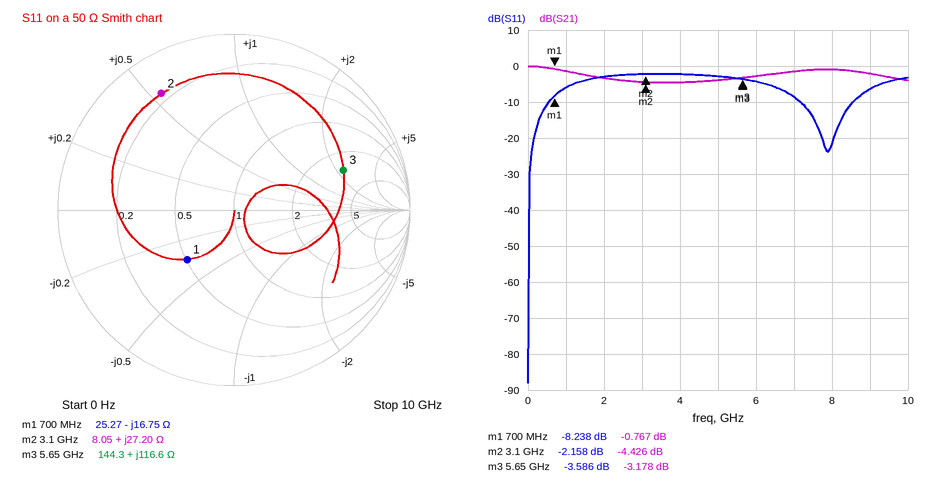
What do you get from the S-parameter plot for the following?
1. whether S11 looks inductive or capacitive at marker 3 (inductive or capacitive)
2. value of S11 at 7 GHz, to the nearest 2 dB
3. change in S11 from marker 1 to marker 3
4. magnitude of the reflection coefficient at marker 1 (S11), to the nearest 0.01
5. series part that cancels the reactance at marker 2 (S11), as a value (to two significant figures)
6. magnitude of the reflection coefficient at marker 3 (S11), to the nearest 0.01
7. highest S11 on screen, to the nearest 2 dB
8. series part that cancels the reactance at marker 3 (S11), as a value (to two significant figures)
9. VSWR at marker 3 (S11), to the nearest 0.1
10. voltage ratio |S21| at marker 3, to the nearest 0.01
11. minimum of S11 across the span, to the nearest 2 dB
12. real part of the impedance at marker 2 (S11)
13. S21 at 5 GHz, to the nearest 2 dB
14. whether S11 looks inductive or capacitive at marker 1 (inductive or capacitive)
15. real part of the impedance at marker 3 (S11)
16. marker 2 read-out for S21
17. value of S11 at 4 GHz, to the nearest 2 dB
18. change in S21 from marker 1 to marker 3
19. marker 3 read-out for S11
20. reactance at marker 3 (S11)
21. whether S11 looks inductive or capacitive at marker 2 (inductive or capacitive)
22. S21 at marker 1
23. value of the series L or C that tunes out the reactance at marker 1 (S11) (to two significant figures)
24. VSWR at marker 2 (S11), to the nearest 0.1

inductive
-8 dB
4.652 dB
0.39
1.9 pF
0.66
-2 dB
240 fF
4.9
0.69
-88 dB
8.05 Ω
-4 dB
capacitive
144.3 Ω
-4.426 dB
-2 dB
-2.411 dB
-3.586 dB
+116.6 Ω
inductive
-0.767 dB
3.8 nH
8.1
